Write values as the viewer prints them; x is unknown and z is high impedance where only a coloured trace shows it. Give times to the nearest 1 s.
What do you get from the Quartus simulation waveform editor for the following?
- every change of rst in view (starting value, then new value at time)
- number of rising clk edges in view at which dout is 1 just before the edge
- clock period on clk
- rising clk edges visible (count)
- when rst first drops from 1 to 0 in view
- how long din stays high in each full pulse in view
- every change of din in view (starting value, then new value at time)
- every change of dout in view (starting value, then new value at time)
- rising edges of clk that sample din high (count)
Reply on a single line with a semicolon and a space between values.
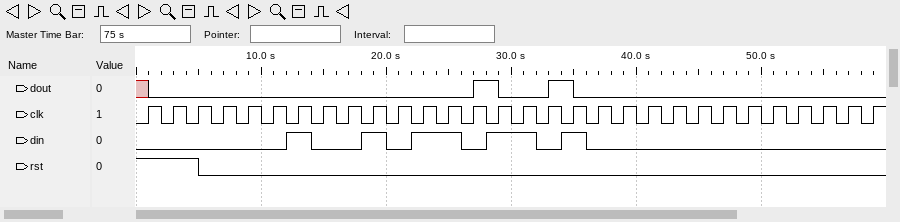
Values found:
1, 0 at 5 s; 2; 2 s; 30; 5 s; 2 s, 2 s, 4 s, 4 s, 2 s; 0, 1 at 12 s, 0 at 14 s, 1 at 18 s, 0 at 20 s, 1 at 22 s, 0 at 26 s, 1 at 28 s, 0 at 32 s, 1 at 34 s, 0 at 36 s; x, 0 at 1 s, 1 at 27 s, 0 at 29 s, 1 at 33 s, 0 at 35 s; 7
